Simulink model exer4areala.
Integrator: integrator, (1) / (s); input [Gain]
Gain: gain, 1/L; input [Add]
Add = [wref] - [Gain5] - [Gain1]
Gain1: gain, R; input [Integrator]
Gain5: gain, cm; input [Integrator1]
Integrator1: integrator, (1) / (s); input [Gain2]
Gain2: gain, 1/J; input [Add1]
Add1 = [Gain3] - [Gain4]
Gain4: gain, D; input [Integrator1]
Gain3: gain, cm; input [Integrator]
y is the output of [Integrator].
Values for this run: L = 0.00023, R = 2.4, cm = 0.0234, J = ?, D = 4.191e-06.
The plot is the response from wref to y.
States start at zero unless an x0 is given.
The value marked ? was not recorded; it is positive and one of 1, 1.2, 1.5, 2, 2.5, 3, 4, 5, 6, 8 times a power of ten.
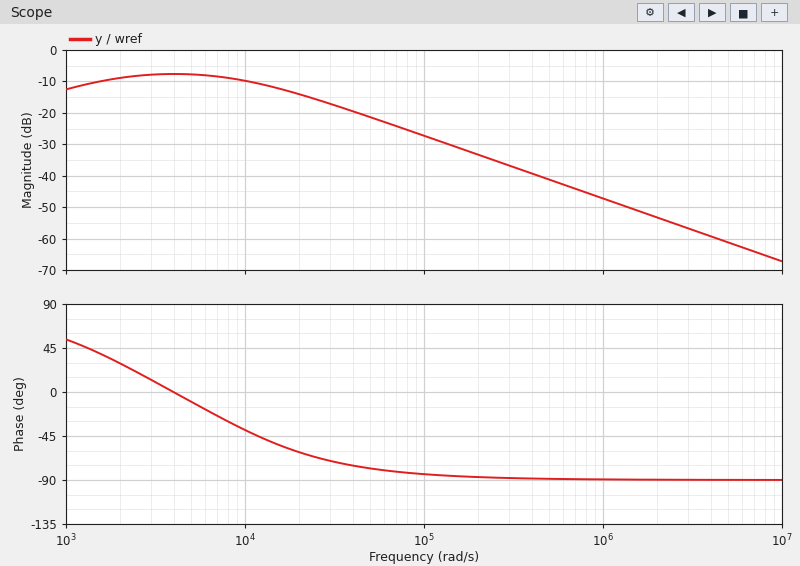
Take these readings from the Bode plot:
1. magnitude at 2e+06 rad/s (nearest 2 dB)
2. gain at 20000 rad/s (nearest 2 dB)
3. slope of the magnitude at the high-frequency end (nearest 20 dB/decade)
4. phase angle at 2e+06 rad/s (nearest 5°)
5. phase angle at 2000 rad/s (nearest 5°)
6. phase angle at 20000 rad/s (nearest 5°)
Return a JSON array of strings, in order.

["-54 dB", "-14 dB", "-20 dB/decade", "-90°", "30°", "-60°"]
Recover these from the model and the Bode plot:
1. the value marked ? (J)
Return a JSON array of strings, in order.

["1.5e-07"]
